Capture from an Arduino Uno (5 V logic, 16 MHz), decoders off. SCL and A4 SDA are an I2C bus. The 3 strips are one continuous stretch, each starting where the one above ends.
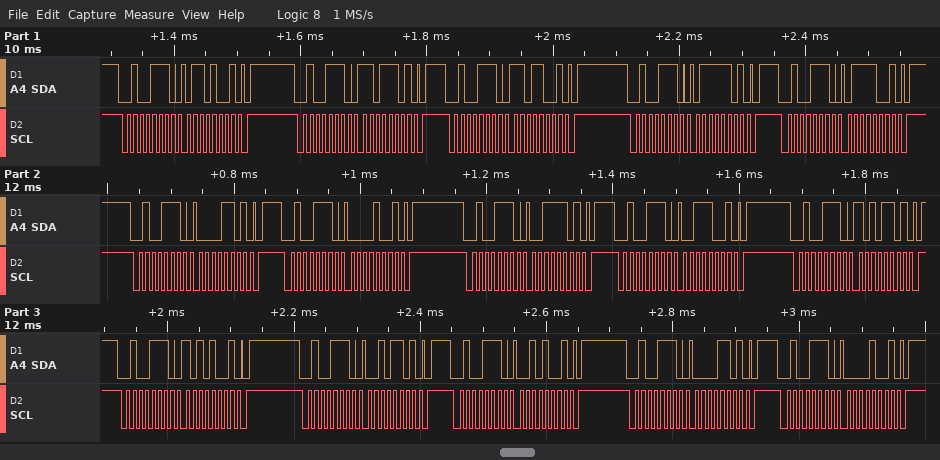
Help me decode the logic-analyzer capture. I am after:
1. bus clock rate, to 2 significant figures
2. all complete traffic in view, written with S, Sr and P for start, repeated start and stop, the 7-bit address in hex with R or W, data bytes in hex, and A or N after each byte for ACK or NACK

100 kHz
S 27W A 69 A P S 27W A DD A P S 27W A D9 A P S 27W A 7D A P S 27W A 79 A P S 27W A 0D A P S 27W A 09 A P S 27W A 3D A P S 27W A 39 A P S 27W A AD A P S 27W A A9 A P S 27W A 2D A P S 27W A 29 A P S 27W A 0D A P S 27W A 09 A P
